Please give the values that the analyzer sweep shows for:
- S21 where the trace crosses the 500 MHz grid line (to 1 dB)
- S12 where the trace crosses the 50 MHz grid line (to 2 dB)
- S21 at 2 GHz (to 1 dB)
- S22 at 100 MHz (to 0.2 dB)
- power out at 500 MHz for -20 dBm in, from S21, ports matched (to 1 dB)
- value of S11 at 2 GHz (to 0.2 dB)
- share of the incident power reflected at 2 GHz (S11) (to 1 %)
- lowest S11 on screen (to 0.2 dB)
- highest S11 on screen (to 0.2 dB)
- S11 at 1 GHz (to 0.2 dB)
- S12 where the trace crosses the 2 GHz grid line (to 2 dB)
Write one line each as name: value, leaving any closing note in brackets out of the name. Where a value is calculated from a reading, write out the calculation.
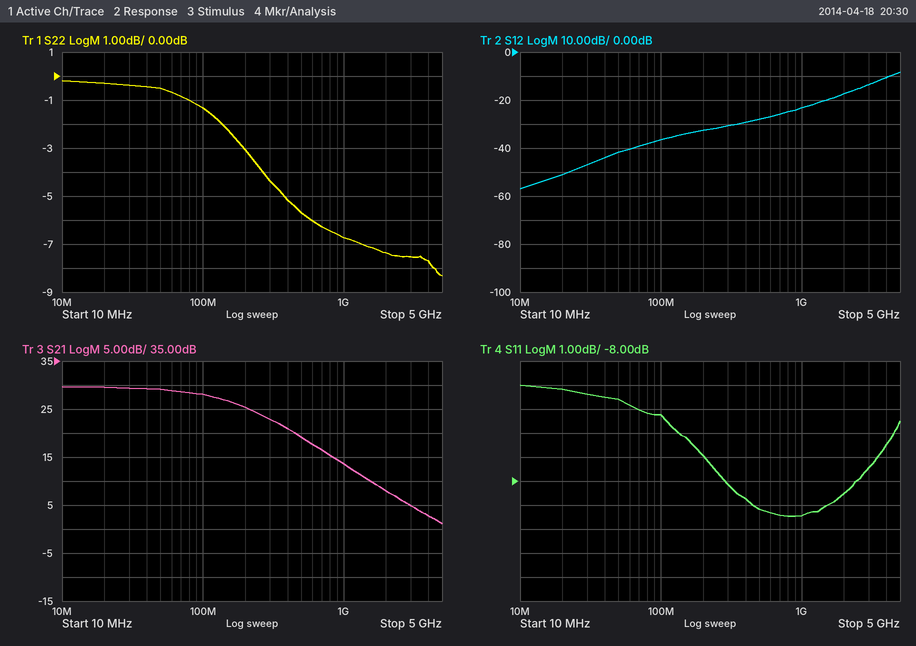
S21 where the trace crosses the 500 MHz grid line: 19 dB
S12 where the trace crosses the 50 MHz grid line: -42 dB
S21 at 2 GHz: 8 dB
S22 at 100 MHz: -1.4 dB
power out at 500 MHz for -20 dBm in, from S21, ports matched: -20 dBm + (19 dB) = -1 dBm
value of S11 at 2 GHz: -8.6 dB
share of the incident power reflected at 2 GHz (S11): 10^(-8.6/10) ≈ 14 %
lowest S11 on screen: -9.4 dB
highest S11 on screen: -4.0 dB
S11 at 1 GHz: -9.4 dB
S12 where the trace crosses the 2 GHz grid line: -18 dB
